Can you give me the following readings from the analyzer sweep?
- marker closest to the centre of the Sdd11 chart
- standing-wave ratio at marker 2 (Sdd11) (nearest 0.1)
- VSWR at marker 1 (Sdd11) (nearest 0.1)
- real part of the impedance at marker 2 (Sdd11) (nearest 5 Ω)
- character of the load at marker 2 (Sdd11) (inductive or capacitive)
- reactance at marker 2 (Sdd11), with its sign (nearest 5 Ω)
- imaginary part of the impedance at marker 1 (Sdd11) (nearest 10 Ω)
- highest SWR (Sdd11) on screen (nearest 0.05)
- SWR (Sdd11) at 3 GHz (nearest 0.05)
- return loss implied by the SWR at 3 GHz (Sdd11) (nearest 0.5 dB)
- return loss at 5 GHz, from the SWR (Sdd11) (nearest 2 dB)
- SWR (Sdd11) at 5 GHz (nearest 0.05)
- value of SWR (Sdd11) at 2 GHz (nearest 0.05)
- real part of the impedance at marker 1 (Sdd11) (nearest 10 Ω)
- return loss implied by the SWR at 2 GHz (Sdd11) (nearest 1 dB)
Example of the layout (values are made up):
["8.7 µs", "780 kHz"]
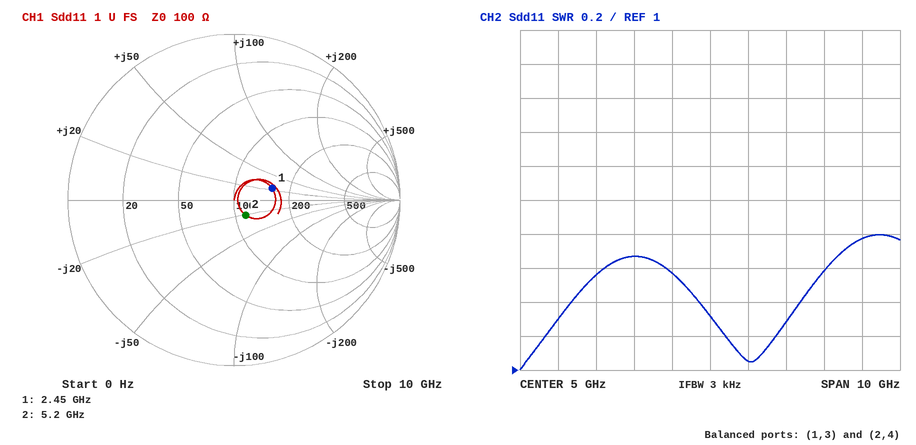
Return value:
["marker 2", "1.3", "1.6", "115 Ω", "capacitive", "-20 Ω", "+20 Ω", "1.80", "1.65", "12.0 dB", "18 dB", "1.30", "1.55", "160 Ω", "13 dB"]
